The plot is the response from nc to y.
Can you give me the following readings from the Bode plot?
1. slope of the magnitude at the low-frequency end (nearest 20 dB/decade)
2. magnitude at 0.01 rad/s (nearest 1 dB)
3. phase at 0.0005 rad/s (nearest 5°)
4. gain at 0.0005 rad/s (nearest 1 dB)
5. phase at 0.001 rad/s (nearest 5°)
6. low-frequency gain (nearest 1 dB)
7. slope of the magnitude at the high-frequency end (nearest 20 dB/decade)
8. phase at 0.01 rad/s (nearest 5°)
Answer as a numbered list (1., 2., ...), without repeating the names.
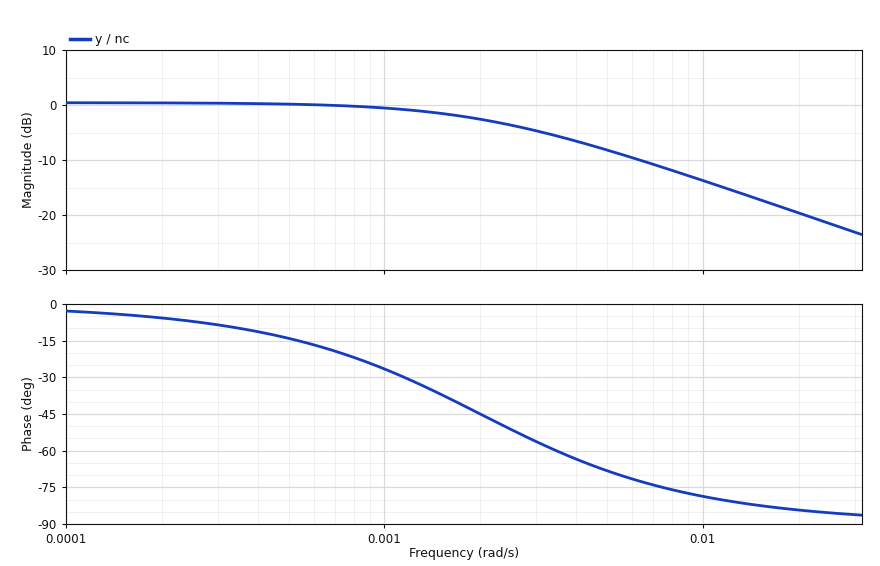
1. 0 dB/decade
2. -14 dB
3. -15°
4. 0 dB
5. -25°
6. 0 dB
7. -20 dB/decade
8. -80°
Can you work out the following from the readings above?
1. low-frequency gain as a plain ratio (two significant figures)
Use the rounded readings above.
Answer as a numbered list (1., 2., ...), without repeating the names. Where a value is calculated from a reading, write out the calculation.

1. 10^(0 / 20) = 1.0
